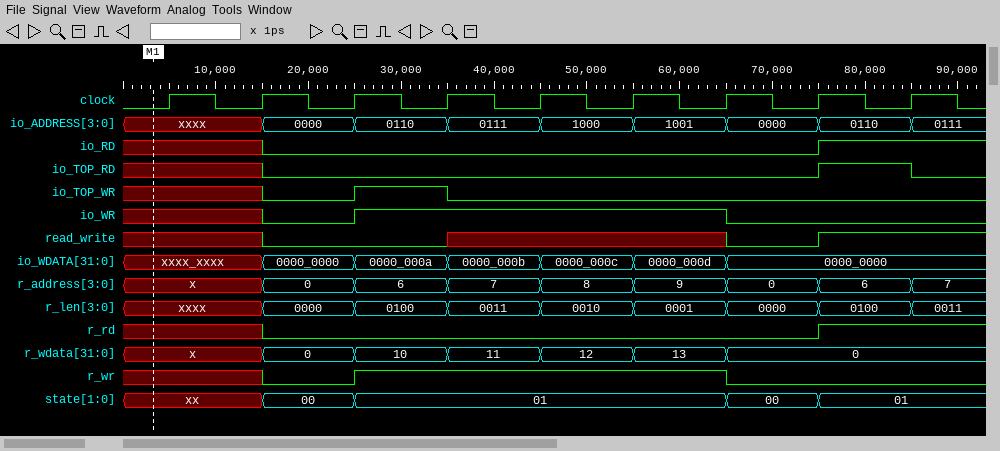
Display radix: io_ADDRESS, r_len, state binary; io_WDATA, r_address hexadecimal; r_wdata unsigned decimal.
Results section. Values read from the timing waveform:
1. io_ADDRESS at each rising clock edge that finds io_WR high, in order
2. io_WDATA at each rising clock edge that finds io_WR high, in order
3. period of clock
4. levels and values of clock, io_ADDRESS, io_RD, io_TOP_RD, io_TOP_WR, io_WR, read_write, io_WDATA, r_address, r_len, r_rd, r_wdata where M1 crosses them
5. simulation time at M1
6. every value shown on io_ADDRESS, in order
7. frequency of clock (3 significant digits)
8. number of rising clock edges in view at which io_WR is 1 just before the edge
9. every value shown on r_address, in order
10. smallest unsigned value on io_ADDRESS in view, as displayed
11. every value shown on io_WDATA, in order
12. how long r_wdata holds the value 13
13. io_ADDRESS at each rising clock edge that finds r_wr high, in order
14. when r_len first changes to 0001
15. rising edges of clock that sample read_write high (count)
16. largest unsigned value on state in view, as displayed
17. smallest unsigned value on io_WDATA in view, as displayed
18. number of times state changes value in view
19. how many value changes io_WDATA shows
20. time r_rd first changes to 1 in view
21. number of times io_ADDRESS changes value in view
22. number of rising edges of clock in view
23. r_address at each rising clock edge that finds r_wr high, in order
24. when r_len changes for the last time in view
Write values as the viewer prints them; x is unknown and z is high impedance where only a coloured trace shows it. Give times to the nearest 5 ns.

0110, 0111, 1000, 1001
0000_000a, 0000_000b, 0000_000c, 0000_000d
10 ns
clock=0, io_ADDRESS=xxxx, io_RD=x, io_TOP_RD=x, io_TOP_WR=x, io_WR=x, read_write=x, io_WDATA=xxxx_xxxx, r_address=x, r_len=xxxx, r_rd=x, r_wdata=x
5 ns
xxxx, 0000, 0110, 0111, 1000, 1001, 0000, 0110, 0111
100 MHz
4
x, 0, 6, 7, 8, 9, 0, 6, 7
0000
xxxx_xxxx, 0000_0000, 0000_000a, 0000_000b, 0000_000c, 0000_000d, 0000_0000
10 ns
0110, 0111, 1000, 1001
55 ns
1
01
0000_0000
4
6
75 ns
8
9
6, 7, 8, 9
85 ns
